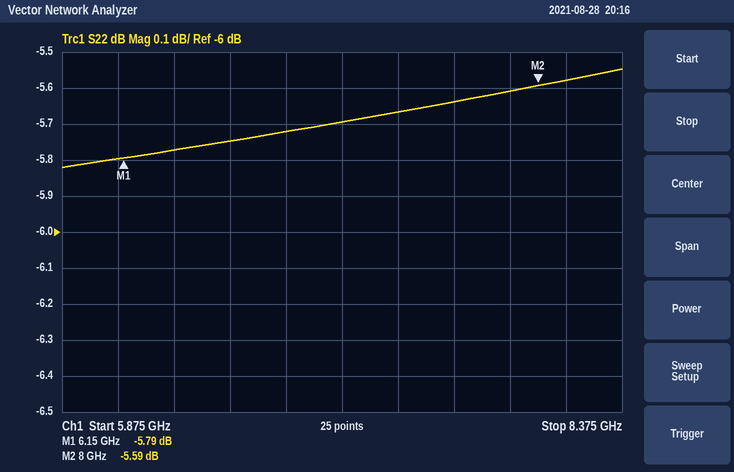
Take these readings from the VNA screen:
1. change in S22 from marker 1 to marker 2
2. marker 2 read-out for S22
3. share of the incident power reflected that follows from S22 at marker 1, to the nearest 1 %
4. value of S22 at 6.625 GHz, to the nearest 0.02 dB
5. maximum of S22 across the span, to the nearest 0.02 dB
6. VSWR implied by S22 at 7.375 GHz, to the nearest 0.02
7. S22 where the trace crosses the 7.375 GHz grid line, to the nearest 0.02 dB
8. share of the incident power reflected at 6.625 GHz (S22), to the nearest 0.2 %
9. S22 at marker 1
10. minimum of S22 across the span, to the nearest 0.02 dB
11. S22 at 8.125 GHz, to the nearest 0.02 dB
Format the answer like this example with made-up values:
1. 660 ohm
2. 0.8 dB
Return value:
1. 0.20 dB
2. -5.59 dB
3. 26 %
4. -5.74 dB
5. -5.54 dB
6. 3.18
7. -5.66 dB
8. 26.6 %
9. -5.79 dB
10. -5.82 dB
11. -5.58 dB
